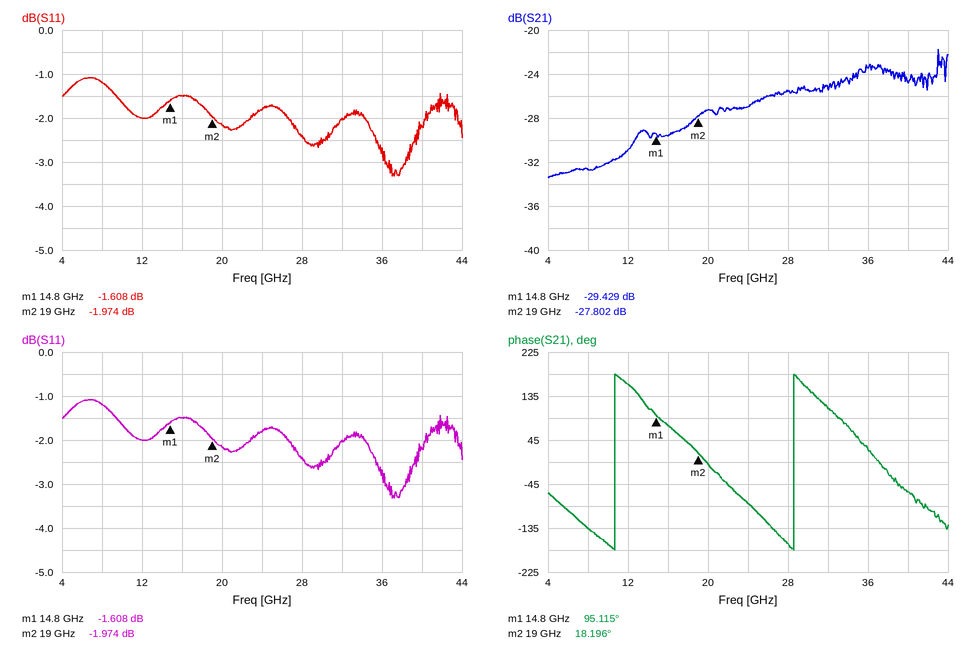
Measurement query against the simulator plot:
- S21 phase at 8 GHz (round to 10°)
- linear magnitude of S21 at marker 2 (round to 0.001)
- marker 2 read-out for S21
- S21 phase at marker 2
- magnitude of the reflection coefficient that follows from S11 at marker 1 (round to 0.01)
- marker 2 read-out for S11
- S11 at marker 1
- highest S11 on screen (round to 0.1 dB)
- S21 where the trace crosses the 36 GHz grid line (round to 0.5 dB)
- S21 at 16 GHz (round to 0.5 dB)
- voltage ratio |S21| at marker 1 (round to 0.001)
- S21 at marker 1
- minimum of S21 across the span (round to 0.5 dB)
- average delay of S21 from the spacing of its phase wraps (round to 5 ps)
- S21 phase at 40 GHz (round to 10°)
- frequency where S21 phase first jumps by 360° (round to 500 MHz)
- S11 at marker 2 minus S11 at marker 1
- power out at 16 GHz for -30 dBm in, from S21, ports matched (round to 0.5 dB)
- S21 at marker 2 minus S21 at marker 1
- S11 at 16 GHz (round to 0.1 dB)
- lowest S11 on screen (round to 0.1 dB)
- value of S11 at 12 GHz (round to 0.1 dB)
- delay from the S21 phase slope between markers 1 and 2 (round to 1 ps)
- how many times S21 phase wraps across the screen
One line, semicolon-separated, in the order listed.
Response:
-140°; 0.041; -27.802 dB; 18.196°; 0.83; -1.974 dB; -1.608 dB; -1.1 dB; -23.5 dB; -29.5 dB; 0.034; -29.429 dB; -33.5 dB; 55 ps; -60°; 10.5 GHz; -0.366 dB; -59.5 dBm; 1.627 dB; -1.5 dB; -3.3 dB; -2.0 dB; 51 ps; 2
